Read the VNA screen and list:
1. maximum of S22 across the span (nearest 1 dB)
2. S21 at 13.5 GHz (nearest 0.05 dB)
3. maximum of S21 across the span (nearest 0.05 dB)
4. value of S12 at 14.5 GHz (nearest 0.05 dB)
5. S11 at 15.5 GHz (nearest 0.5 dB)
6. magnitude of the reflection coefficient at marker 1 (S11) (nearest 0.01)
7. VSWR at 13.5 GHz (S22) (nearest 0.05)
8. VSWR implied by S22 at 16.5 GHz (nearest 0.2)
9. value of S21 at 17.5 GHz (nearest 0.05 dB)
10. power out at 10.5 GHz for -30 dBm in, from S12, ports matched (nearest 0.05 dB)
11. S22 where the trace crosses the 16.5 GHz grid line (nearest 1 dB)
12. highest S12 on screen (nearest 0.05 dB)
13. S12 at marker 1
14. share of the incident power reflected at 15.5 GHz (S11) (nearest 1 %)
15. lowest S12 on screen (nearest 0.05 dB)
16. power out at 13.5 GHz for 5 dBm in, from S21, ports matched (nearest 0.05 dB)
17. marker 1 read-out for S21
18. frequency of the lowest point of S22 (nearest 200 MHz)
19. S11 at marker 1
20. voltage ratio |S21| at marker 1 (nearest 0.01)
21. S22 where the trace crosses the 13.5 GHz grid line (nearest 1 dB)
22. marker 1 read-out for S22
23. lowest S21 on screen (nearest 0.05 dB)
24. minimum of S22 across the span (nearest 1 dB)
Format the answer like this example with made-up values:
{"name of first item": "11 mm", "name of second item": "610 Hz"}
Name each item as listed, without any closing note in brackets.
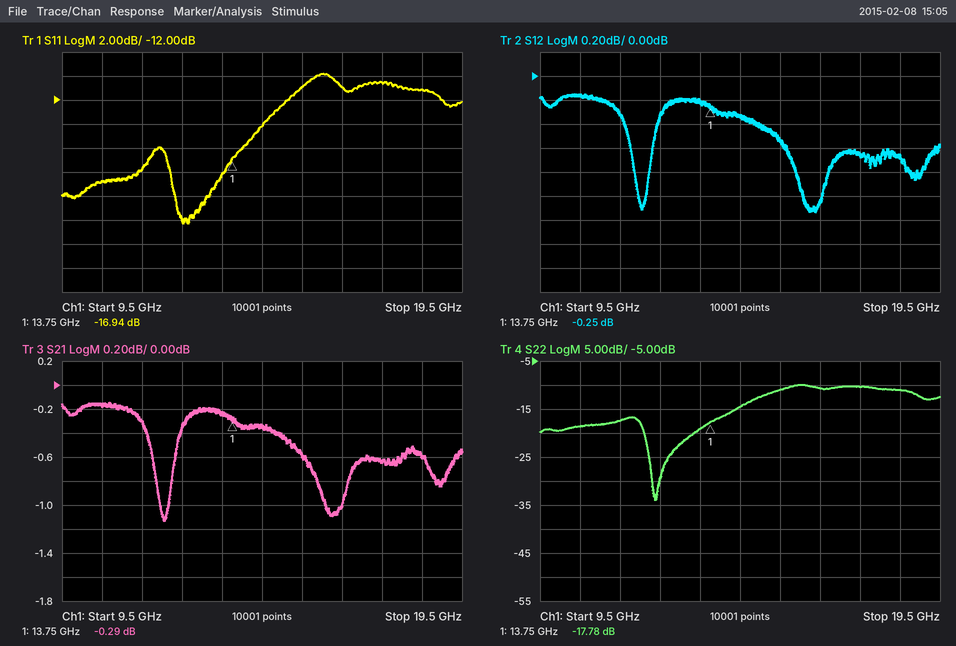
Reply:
{"maximum of S22 across the span": "-10 dB", "S21 at 13.5 GHz": "-0.25 dB", "maximum of S21 across the span": "-0.15 dB", "value of S12 at 14.5 GHz": "-0.35 dB", "S11 at 15.5 GHz": "-11.0 dB", "magnitude of the reflection coefficient at marker 1 (S11)": "0.14", "VSWR at 13.5 GHz (S22)": "1.25", "VSWR implied by S22 at 16.5 GHz": "1.8", "value of S21 at 17.5 GHz": "-0.65 dB", "power out at 10.5 GHz for -30 dBm in, from S12, ports matched": "-30.15 dBm", "S22 where the trace crosses the 16.5 GHz grid line": "-11 dB", "highest S12 on screen": "-0.15 dB", "S12 at marker 1": "-0.25 dB", "share of the incident power reflected at 15.5 GHz (S11)": "8 %", "lowest S12 on screen": "-1.15 dB", "power out at 13.5 GHz for 5 dBm in, from S21, ports matched": "4.75 dBm", "marker 1 read-out for S21": "-0.29 dB", "frequency of the lowest point of S22": "12.4 GHz", "S11 at marker 1": "-16.94 dB", "voltage ratio |S21| at marker 1": "0.97", "S22 where the trace crosses the 13.5 GHz grid line": "-19 dB", "marker 1 read-out for S22": "-17.78 dB", "lowest S21 on screen": "-1.15 dB", "minimum of S22 across the span": "-34 dB"}
